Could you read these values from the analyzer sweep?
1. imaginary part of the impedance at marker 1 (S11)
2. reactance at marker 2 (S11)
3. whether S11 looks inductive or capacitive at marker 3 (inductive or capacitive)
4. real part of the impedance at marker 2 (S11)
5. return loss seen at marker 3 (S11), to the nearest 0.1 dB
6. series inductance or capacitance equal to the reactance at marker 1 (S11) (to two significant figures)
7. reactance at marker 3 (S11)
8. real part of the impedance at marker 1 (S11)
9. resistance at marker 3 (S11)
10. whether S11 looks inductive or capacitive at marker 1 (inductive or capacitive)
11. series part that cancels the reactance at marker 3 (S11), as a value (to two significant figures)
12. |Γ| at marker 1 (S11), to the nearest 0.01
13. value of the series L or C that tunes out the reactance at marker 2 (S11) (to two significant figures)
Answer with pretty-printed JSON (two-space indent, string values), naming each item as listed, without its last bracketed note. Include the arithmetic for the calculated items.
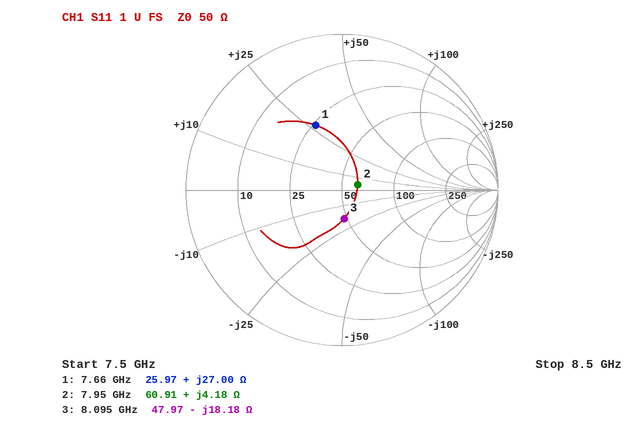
{
  "imaginary part of the impedance at marker 1": "+27.00 Ω",
  "reactance at marker 2": "+4.18 Ω",
  "whether S11 looks inductive or capacitive at marker 3": "capacitive",
  "real part of the impedance at marker 2": "60.91 Ω",
  "return loss seen at marker 3 (S11), to the nearest 0.1 dB": "14.7 dB",
  "series inductance or capacitance equal to the reactance at marker 1 (S11)": "L = 27 Ω/(2π × 7.66 GHz) ≈ 561 pH, so 560 pH to two significant figures",
  "reactance at marker 3": "-18.18 Ω",
  "real part of the impedance at marker 1": "25.97 Ω",
  "resistance at marker 3": "47.97 Ω",
  "whether S11 looks inductive or capacitive at marker 1": "inductive",
  "series part that cancels the reactance at marker 3 (S11), as a value": "L = 18.18 Ω/(2π × 8.095 GHz) ≈ 357 pH, so 360 pH to two significant figures",
  "|Γ| at marker 1 (S11), to the nearest 0.01": "0.45",
  "value of the series L or C that tunes out the reactance at marker 2 (S11)": "C = 1/(2π × 7.95 GHz × 4.18 Ω) ≈ 4.8 pF"
}
